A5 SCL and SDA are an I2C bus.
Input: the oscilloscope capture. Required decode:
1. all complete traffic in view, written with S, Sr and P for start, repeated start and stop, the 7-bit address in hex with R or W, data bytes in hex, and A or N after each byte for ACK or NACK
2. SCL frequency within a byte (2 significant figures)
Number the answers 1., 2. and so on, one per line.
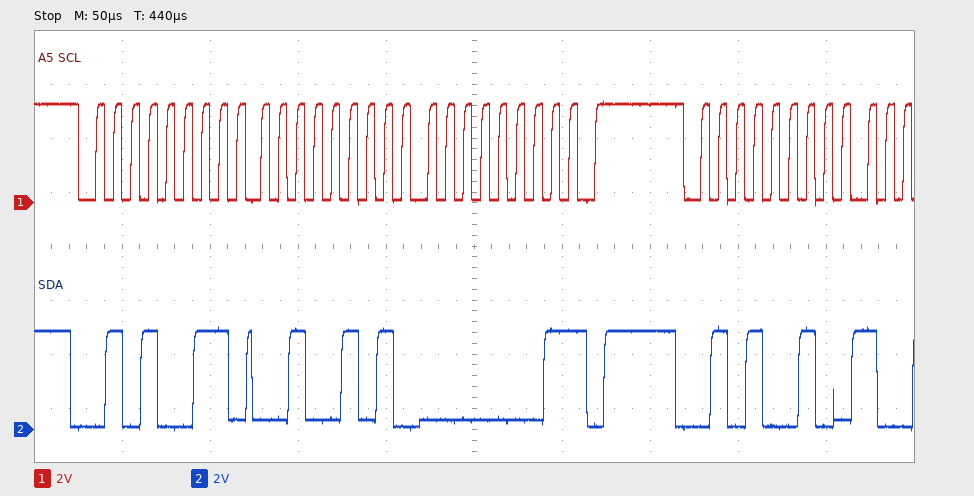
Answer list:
1. S 29R A 25 A 01 N P S 29W A
2. 100 kHz
